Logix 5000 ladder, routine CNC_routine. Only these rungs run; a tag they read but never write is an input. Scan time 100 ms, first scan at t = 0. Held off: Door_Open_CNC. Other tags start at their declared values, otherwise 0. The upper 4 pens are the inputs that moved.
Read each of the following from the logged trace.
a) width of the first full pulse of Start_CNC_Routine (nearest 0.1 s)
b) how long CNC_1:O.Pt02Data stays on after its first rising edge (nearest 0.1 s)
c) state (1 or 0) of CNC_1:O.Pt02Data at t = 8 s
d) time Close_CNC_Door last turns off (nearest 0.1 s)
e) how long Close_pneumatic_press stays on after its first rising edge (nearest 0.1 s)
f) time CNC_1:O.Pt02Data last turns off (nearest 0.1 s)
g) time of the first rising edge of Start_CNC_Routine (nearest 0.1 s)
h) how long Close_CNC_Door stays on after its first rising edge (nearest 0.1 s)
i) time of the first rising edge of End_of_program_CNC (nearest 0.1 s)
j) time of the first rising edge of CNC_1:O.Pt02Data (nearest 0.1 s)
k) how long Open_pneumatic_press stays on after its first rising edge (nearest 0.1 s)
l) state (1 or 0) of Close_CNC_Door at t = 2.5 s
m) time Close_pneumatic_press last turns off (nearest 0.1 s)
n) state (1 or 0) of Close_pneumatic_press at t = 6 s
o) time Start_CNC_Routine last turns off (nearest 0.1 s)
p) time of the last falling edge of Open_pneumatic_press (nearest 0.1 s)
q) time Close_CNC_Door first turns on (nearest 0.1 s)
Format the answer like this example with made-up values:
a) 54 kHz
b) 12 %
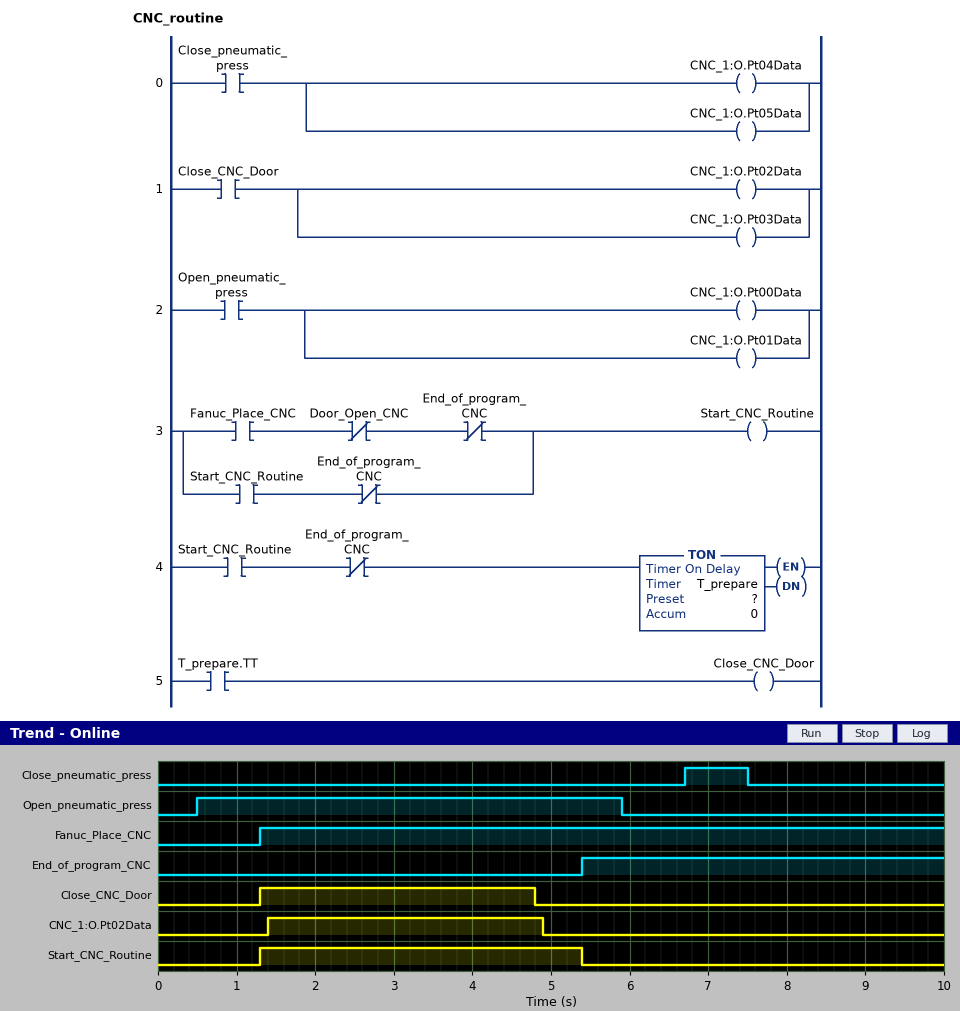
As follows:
a) 4.1 s
b) 3.5 s
c) 0
d) 4.8 s
e) 0.8 s
f) 4.9 s
g) 1.3 s
h) 3.5 s
i) 5.4 s
j) 1.4 s
k) 5.4 s
l) 1
m) 7.5 s
n) 0
o) 5.4 s
p) 5.9 s
q) 1.3 s
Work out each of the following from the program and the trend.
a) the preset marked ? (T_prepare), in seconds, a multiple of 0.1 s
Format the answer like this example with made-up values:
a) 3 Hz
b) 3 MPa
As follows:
a) 3.5 s
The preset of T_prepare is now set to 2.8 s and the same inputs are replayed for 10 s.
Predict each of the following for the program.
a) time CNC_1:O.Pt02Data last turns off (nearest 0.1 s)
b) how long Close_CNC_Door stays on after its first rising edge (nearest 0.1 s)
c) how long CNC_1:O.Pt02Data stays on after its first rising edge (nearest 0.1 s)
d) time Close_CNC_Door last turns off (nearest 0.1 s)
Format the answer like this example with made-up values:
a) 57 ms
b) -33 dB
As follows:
a) 4.2 s
b) 2.8 s
c) 2.8 s
d) 4.1 s
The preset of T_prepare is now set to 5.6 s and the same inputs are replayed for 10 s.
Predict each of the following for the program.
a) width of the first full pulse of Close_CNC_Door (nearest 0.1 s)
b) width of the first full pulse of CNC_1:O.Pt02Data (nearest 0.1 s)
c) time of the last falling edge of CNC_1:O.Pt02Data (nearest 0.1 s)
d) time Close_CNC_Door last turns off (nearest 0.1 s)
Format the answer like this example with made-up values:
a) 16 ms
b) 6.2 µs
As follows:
a) 4.1 s
b) 4.1 s
c) 5.5 s
d) 5.4 s
